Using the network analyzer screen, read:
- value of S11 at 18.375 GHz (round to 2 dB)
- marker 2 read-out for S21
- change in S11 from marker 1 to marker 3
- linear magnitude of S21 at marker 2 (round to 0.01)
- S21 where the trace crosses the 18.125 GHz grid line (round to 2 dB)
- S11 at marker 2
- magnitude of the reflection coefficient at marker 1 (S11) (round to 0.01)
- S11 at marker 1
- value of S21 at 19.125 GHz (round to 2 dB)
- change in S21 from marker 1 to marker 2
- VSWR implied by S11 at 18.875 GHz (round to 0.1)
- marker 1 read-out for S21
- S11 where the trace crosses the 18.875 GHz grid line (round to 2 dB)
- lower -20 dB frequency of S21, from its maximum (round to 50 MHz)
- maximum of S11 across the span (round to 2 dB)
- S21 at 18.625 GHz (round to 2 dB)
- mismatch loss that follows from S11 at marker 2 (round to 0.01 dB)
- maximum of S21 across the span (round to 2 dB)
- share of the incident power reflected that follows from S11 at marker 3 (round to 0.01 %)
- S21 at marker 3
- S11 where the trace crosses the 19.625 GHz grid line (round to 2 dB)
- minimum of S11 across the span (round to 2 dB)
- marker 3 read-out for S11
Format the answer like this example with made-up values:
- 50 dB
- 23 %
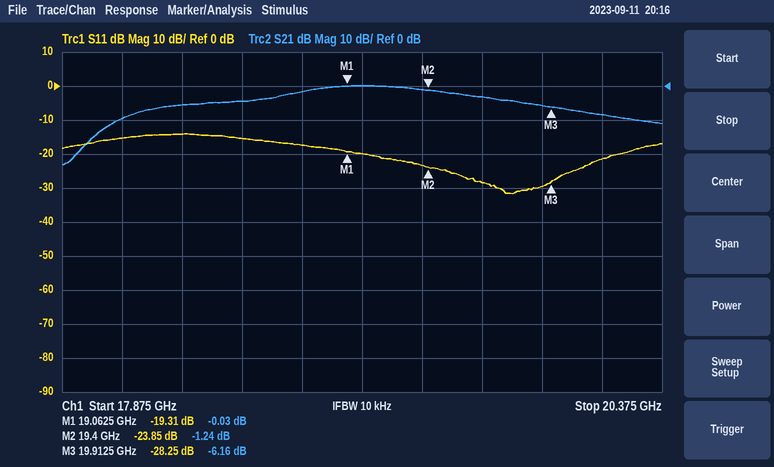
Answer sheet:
- -14 dB
- -1.24 dB
- -8.94 dB
- 0.87
- -10 dB
- -23.85 dB
- 0.11
- -19.31 dB
- 0 dB
- -1.21 dB
- 1.3
- -0.03 dB
- -18 dB
- 17.95 GHz
- -14 dB
- -4 dB
- 0.02 dB
- 0 dB
- 0.15 %
- -6.16 dB
- -28 dB
- -32 dB
- -28.25 dB
